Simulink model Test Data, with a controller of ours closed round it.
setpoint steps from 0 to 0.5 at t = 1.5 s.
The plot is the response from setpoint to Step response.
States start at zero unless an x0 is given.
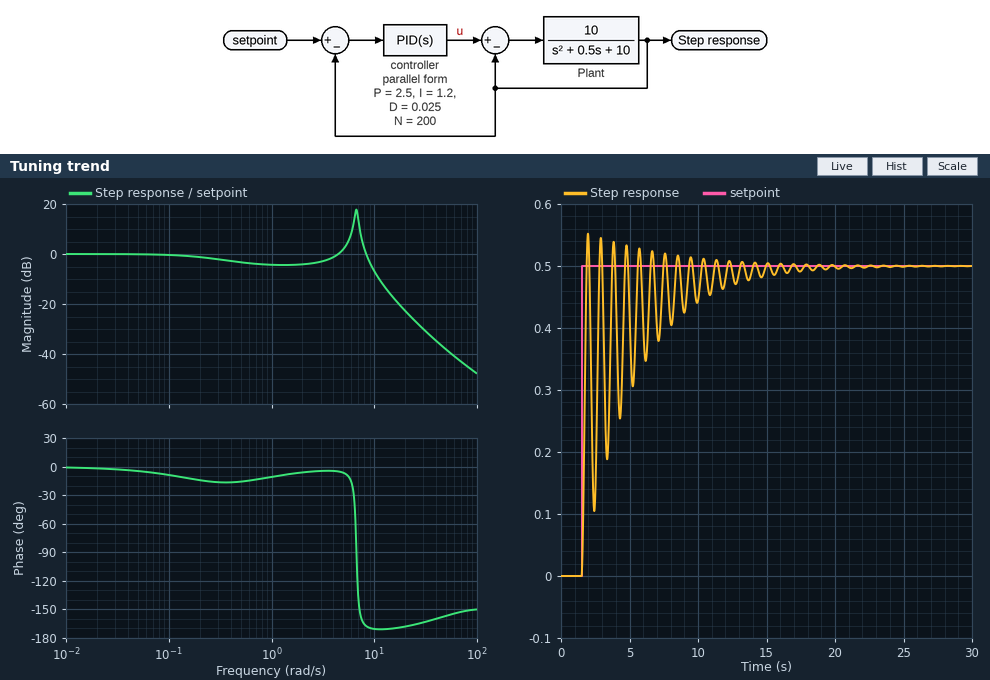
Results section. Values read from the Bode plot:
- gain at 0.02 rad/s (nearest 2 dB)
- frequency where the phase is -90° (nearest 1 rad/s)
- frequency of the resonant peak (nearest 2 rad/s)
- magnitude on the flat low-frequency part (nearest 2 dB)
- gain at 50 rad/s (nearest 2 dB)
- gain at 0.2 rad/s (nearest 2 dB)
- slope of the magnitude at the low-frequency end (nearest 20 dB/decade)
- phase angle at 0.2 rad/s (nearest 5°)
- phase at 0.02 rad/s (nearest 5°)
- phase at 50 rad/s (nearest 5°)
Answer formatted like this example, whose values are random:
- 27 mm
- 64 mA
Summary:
- 0 dB
- 7 rad/s
- 6 rad/s
- 0 dB
- -38 dB
- -2 dB
- 0 dB/decade
- -15°
- 0°
- -155°
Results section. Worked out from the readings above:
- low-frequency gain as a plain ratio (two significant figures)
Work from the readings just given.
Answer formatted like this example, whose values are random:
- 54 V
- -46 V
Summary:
- 1.0
